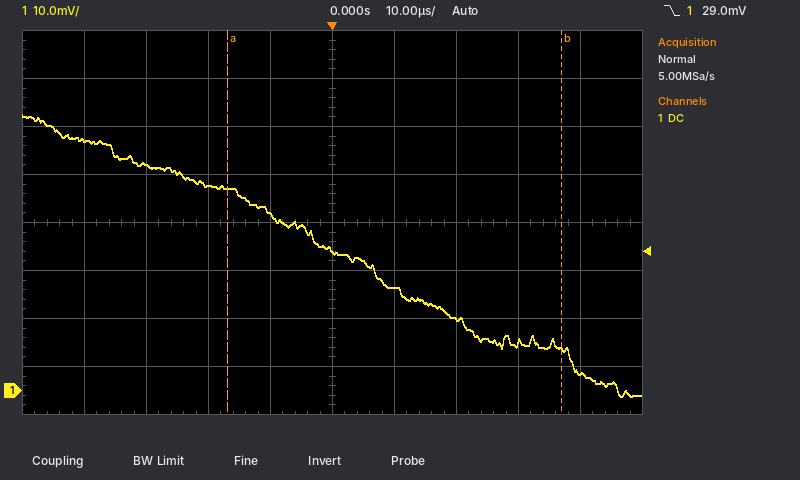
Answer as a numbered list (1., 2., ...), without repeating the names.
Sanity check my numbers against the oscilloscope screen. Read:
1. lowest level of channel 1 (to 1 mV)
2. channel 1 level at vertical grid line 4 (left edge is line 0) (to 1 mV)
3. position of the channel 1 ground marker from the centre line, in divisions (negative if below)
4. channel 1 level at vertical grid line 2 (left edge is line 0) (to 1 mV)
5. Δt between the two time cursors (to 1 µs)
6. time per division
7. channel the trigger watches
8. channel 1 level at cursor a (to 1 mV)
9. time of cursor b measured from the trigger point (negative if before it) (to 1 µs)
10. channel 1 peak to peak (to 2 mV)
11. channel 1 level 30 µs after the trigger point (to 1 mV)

1. -1 mV
2. 37 mV
3. -3.5 div
4. 47 mV
5. 54 µs
6. 10 µs
7. channel 1
8. 42 mV
9. +37 µs
10. 58 mV
11. 10 mV
